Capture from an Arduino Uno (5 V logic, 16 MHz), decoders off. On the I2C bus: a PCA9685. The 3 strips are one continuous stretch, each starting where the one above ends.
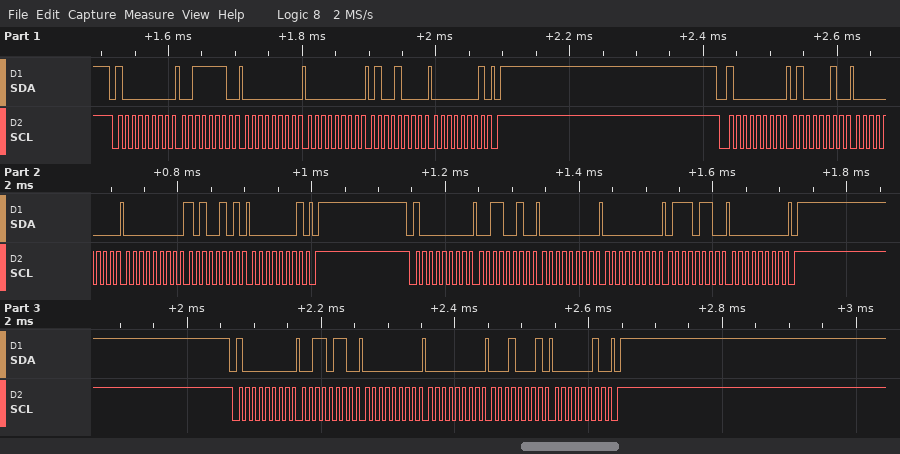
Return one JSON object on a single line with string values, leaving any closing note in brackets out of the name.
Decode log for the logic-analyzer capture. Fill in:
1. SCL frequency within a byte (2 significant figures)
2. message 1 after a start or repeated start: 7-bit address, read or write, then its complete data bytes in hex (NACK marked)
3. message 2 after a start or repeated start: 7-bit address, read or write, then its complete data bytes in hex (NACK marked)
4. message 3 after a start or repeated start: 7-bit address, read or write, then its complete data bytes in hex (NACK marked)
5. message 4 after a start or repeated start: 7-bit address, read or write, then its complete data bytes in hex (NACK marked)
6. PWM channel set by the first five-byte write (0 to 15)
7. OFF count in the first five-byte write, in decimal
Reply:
{"SCL frequency within a byte": "100 kHz", "message 1 after a start or repeated start: 7-bit address, read or write, then its complete data bytes in hex": "0x40 write: 3E 00 00 48 01", "message 2 after a start or repeated start: 7-bit address, read or write, then its complete data bytes in hex": "0x40 write: 42 00 00 A5 01", "message 3 after a start or repeated start: 7-bit address, read or write, then its complete data bytes in hex": "0x40 write: 32 00 00 76 00", "message 4 after a start or repeated start: 7-bit address, read or write, then its complete data bytes in hex": "0x40 write: 36 00 00 11 02", "PWM channel set by the first five-byte write": "14", "OFF count in the first five-byte write, in decimal": "328"}
